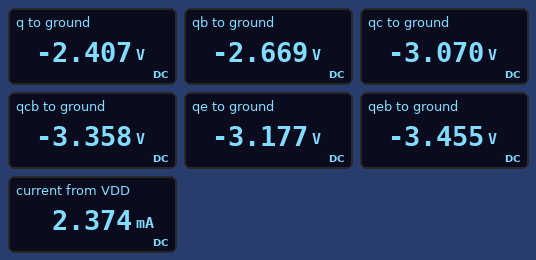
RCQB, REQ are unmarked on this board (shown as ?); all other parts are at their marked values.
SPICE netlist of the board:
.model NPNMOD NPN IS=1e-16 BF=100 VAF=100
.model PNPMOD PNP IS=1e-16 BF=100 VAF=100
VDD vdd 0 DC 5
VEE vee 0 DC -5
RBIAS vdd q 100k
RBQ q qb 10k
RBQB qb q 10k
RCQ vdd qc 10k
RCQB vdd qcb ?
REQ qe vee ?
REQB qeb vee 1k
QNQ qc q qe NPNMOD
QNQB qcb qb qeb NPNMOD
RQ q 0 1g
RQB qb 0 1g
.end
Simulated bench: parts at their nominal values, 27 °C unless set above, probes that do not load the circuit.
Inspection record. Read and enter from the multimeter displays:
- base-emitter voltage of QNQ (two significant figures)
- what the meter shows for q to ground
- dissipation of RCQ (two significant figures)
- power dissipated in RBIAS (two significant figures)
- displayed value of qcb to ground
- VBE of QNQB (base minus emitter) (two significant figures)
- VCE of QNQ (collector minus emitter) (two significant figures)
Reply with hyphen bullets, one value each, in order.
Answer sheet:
- 770 mV
- -2.407 V
- 6.5 mW
- 550 µW
- -3.358 V
- 790 mV
- 110 mV
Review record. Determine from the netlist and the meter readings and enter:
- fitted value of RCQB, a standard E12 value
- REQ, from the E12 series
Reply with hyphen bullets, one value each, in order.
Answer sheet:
- 5.6 kΩ
- 2.2 kΩ
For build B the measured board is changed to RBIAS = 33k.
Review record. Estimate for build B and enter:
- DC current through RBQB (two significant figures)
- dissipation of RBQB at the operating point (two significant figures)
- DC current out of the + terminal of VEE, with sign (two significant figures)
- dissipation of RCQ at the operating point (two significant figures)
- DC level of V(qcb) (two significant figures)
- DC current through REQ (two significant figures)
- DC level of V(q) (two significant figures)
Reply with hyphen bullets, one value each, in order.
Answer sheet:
- 44 µA
- 19 µW
- -2.5 mA
- 6.3 mW
- -3.3 V
- 920 µA
- -2.2 V
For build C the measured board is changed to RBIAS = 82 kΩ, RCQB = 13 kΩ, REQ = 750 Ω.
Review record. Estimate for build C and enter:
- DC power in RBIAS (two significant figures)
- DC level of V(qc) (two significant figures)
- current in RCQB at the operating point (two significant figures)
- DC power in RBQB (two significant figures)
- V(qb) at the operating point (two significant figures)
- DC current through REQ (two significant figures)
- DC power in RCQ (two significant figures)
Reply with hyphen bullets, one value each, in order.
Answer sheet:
- 870 µW
- -4.2 V
- 700 µA
- 290 nW
- -3.5 V
- 1.0 mA
- 8.4 mW
